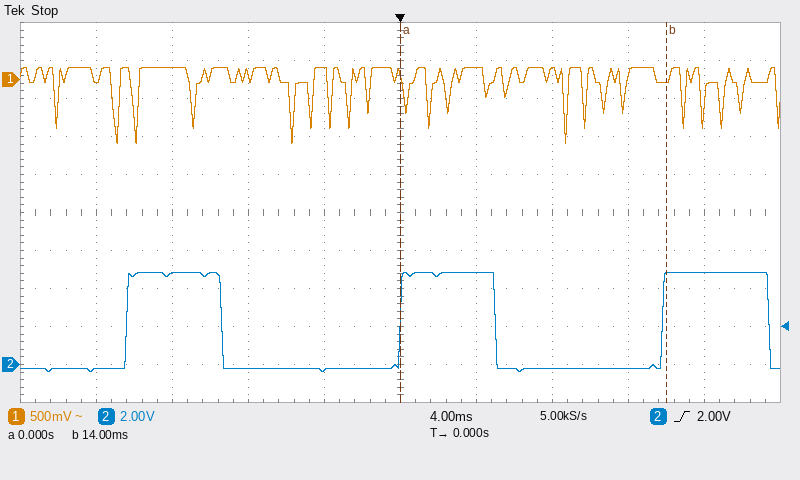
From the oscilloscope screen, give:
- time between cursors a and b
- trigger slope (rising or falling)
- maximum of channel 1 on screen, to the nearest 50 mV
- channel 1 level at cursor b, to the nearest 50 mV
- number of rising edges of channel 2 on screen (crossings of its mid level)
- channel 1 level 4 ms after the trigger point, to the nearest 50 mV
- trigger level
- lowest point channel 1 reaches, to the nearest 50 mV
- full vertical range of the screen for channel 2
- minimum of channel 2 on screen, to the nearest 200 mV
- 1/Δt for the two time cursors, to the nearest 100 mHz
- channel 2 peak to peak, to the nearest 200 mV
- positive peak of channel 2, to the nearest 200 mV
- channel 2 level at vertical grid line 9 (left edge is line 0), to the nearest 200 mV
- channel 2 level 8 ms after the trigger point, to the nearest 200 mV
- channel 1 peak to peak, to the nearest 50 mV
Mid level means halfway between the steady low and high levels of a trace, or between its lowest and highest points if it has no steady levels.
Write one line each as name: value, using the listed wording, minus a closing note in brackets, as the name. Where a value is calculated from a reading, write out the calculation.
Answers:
time between cursors a and b: 14 ms − (0 s) = 14.0 ms
trigger slope: rising
maximum of channel 1 on screen, to the nearest 50 mV: 150 mV
channel 1 level at cursor b, to the nearest 50 mV: 0 mV
number of rising edges of channel 2 on screen: 3
channel 1 level 4 ms after the trigger point, to the nearest 50 mV: 150 mV
trigger level: 2.00 V
lowest point channel 1 reaches, to the nearest 50 mV: -850 mV
full vertical range of the screen for channel 2: 20 V
minimum of channel 2 on screen, to the nearest 200 mV: -400 mV
1/Δt for the two time cursors, to the nearest 100 mHz: 1 / 14.0 ms ≈ 71.4 Hz
channel 2 peak to peak, to the nearest 200 mV: 4.8 V − (-400 mV) = 5.2 V
positive peak of channel 2, to the nearest 200 mV: 4.8 V
channel 2 level at vertical grid line 9 (left edge is line 0), to the nearest 200 mV: 4.8 V
channel 2 level 8 ms after the trigger point, to the nearest 200 mV: -200 mV
channel 1 peak to peak, to the nearest 50 mV: 150 mV − (-850 mV) = 1.00 V
